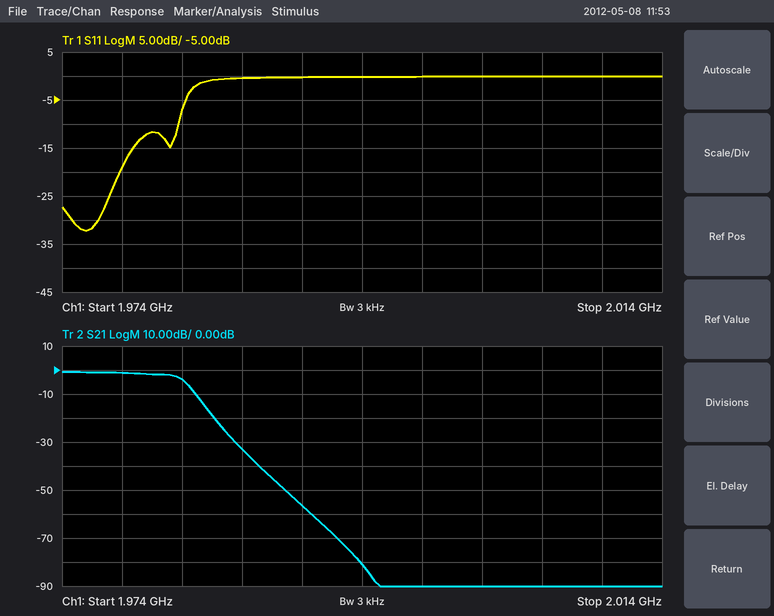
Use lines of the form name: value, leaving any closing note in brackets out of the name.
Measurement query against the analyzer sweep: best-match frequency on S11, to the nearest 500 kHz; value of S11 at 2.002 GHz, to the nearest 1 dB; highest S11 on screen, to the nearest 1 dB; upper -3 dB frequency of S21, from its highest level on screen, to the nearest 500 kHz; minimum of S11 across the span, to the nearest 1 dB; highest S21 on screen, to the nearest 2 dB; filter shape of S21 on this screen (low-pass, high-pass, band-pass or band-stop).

best-match frequency on S11, to the nearest 500 kHz: 1.9755 GHz
value of S11 at 2.002 GHz, to the nearest 1 dB: 0 dB
highest S11 on screen, to the nearest 1 dB: 0 dB
upper -3 dB frequency of S21, from its highest level on screen, to the nearest 500 kHz: 1.9820 GHz
minimum of S11 across the span, to the nearest 1 dB: -32 dB
highest S21 on screen, to the nearest 2 dB: 0 dB
filter shape of S21 on this screen: low-pass
